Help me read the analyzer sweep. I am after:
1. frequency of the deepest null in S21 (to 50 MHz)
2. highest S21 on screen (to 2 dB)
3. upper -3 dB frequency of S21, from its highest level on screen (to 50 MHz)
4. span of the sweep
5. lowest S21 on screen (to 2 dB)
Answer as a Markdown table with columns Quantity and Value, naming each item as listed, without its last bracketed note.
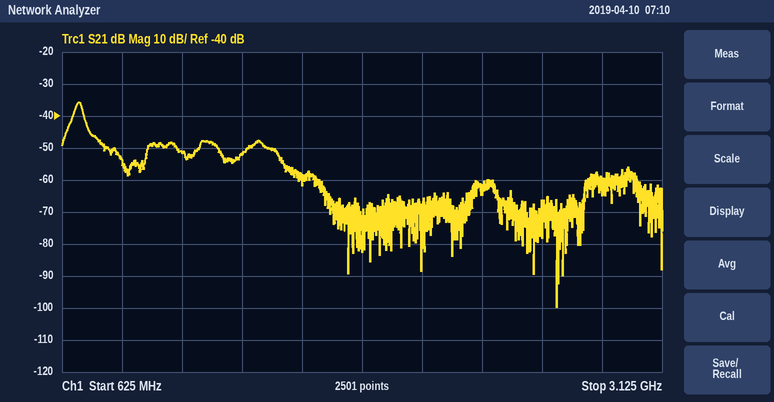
| Quantity | Value |
|---|---|
| frequency of the deepest null in S21 | 2.70 GHz |
| highest S21 on screen | -36 dB |
| upper -3 dB frequency of S21, from its highest level on screen | 700 MHz |
| span of the sweep | 2.5 GHz |
| lowest S21 on screen | -100 dB |
